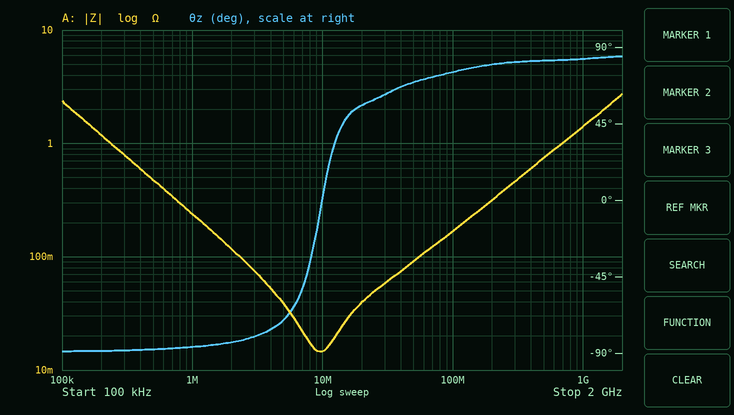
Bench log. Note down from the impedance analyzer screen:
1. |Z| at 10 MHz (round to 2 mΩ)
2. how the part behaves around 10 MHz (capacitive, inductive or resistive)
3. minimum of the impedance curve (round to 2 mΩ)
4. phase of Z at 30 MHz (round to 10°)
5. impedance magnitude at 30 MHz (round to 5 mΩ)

14 mΩ
resistive
14 mΩ
60°
60 mΩ
